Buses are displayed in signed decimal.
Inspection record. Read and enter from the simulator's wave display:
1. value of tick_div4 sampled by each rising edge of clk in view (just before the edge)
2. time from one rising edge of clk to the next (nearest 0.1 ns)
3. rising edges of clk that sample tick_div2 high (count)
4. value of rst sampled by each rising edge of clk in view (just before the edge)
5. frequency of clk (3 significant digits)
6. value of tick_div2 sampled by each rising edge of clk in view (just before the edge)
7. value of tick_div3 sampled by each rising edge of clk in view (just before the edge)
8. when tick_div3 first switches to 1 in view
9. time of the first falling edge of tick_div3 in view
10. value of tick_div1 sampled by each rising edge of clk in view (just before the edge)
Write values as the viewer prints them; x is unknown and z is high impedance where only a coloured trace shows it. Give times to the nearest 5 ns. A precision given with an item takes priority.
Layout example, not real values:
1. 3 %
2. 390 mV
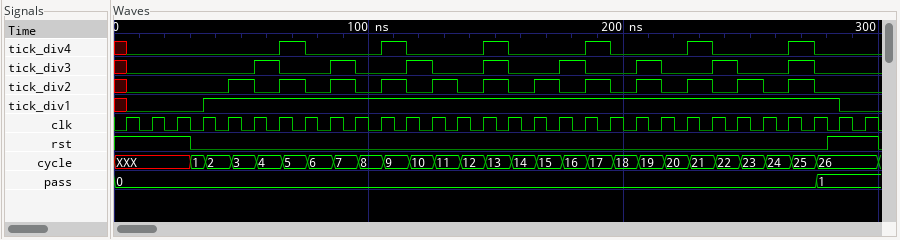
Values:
1. x 0 0 0 0 0 0 1 0 0 0 1 0 0 0 1 0 0 0 1 0 0 0 1 0 0 0 1 0 0
2. 10 ns
3. 12
4. 1 1 1 0 0 0 0 0 0 0 0 0 0 0 0 0 0 0 0 0 0 0 0 0 0 0 0 0 1 1
5. 100 MHz
6. x 0 0 0 0 1 0 1 0 1 0 1 0 1 0 1 0 1 0 1 0 1 0 1 0 1 0 1 0 0
7. x 0 0 0 0 0 1 0 0 1 0 0 1 0 0 1 0 0 1 0 0 1 0 0 1 0 0 1 0 0
8. 55 ns
9. 65 ns
10. x 0 0 0 1 1 1 1 1 1 1 1 1 1 1 1 1 1 1 1 1 1 1 1 1 1 1 1 1 0
